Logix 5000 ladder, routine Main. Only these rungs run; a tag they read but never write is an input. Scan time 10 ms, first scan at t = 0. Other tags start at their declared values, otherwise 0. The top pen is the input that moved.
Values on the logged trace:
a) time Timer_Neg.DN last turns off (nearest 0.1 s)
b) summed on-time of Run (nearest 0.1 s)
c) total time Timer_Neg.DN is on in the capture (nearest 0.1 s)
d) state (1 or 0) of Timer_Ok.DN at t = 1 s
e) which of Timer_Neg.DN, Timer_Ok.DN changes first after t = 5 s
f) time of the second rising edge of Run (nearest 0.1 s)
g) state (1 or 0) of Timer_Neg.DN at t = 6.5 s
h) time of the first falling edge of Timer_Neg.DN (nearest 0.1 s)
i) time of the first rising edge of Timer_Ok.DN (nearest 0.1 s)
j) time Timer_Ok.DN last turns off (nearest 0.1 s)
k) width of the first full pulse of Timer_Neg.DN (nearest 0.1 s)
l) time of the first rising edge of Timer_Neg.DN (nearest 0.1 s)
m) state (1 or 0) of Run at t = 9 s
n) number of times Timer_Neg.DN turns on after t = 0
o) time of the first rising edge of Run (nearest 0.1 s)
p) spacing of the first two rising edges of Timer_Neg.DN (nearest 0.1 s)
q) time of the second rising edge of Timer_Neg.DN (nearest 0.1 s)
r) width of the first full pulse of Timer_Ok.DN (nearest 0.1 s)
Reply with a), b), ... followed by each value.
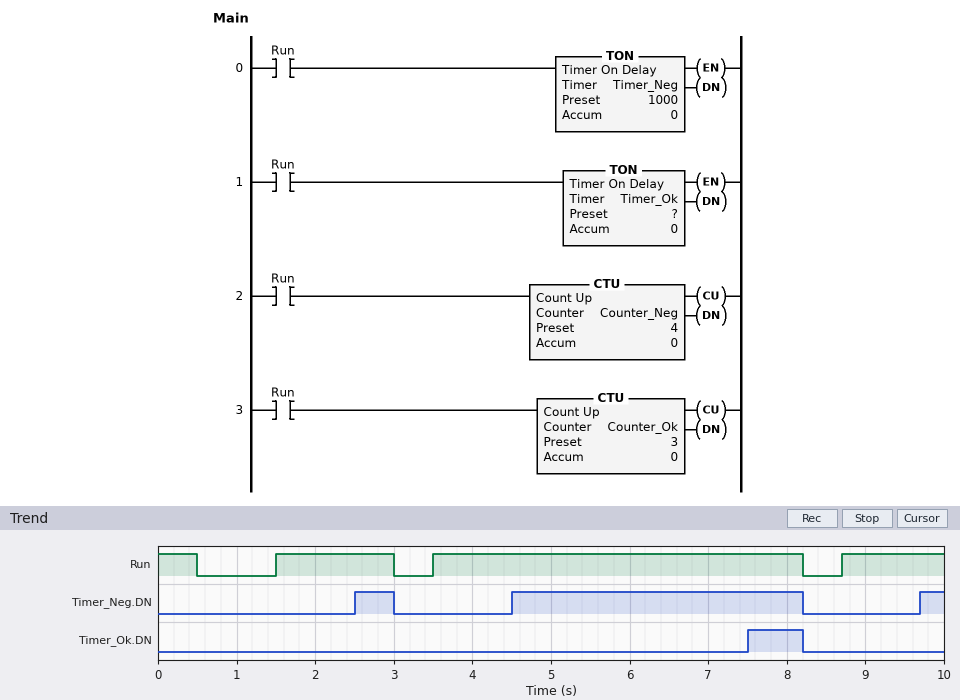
a) 8.2 s
b) 8.0 s
c) 4.5 s
d) 0
e) Timer_Ok.DN
f) 3.5 s
g) 1
h) 3.0 s
i) 7.5 s
j) 8.2 s
k) 0.5 s
l) 2.5 s
m) 1
n) 3
o) 1.5 s
p) 2.0 s
q) 4.5 s
r) 0.7 s
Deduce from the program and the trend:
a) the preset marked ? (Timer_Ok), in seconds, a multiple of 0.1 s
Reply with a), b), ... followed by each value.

a) 4.0 s
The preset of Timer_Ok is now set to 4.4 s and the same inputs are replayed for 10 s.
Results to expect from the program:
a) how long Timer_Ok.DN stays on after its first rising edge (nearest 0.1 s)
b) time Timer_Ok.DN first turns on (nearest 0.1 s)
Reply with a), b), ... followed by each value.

a) 0.3 s
b) 7.9 s
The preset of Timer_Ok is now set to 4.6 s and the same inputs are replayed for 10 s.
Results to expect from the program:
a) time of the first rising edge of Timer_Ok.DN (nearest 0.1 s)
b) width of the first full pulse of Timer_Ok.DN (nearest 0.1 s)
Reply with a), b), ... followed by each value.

a) 8.1 s
b) 0.1 s
